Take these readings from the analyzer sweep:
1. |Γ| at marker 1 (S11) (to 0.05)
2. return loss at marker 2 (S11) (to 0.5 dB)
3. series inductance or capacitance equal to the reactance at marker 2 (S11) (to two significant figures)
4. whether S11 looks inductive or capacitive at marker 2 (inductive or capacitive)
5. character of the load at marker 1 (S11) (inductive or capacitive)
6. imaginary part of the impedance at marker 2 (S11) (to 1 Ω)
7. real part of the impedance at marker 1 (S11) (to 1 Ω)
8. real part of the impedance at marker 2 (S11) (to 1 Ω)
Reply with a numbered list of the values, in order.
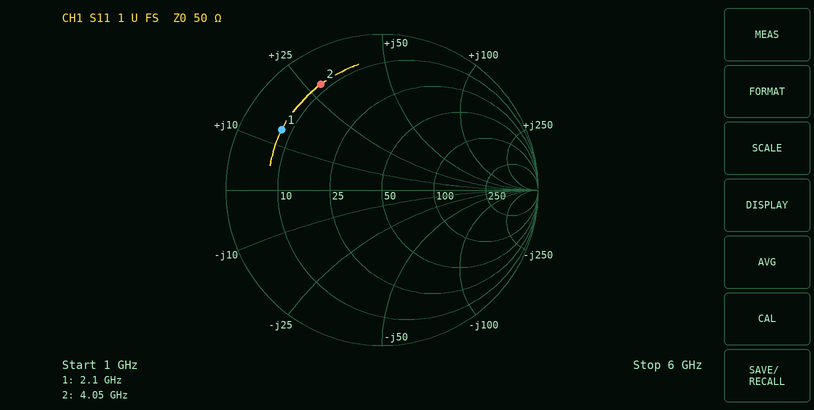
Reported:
1. 0.75
2. 2.0 dB
3. 1.1 nH
4. inductive
5. inductive
6. +28 Ω
7. 8 Ω
8. 8 Ω
